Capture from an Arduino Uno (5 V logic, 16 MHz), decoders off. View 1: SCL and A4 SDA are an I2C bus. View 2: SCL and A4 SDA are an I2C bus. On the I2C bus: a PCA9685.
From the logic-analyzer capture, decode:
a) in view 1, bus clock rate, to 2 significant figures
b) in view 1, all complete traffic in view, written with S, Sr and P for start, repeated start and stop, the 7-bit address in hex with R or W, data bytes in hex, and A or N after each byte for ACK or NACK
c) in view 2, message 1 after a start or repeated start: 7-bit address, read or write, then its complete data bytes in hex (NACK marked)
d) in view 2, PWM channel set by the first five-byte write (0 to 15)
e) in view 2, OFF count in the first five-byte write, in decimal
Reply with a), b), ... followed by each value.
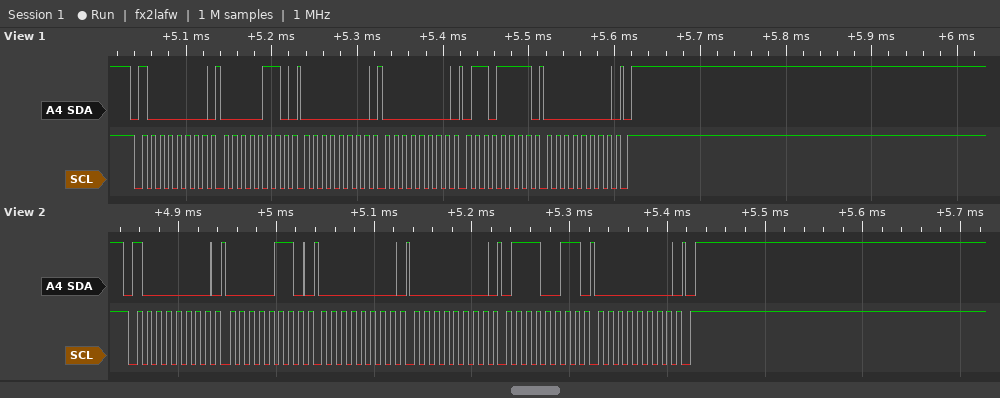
a) 100 kHz
b) S 40W A 06 A 00 A 00 A 6F A 00 A P
c) 0x40 write: 06 00 00 73 00
d) 0
e) 115
